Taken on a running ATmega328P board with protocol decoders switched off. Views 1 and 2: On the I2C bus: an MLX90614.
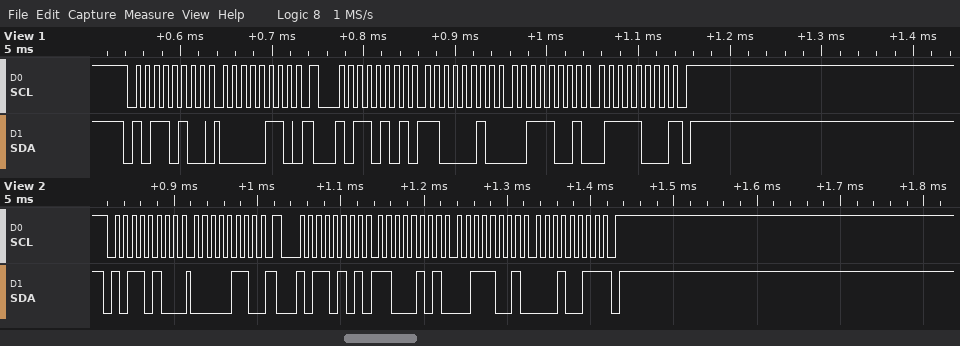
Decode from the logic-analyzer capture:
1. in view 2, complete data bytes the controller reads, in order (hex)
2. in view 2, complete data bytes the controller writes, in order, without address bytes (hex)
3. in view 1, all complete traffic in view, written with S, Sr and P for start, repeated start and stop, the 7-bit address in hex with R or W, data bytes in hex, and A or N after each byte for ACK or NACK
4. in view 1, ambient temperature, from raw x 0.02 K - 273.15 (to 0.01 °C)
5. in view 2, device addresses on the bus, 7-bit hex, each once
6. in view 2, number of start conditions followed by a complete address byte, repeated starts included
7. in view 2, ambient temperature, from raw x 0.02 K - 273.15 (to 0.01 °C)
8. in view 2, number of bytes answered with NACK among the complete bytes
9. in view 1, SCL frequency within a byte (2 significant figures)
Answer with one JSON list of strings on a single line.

["C5 39 13", "06", "S 5AW A 06 A Sr 5AR A C2 A 39 A 78 N P", "22.57 °C", "0x5A", "2", "22.63 °C", "1", "100 kHz"]
